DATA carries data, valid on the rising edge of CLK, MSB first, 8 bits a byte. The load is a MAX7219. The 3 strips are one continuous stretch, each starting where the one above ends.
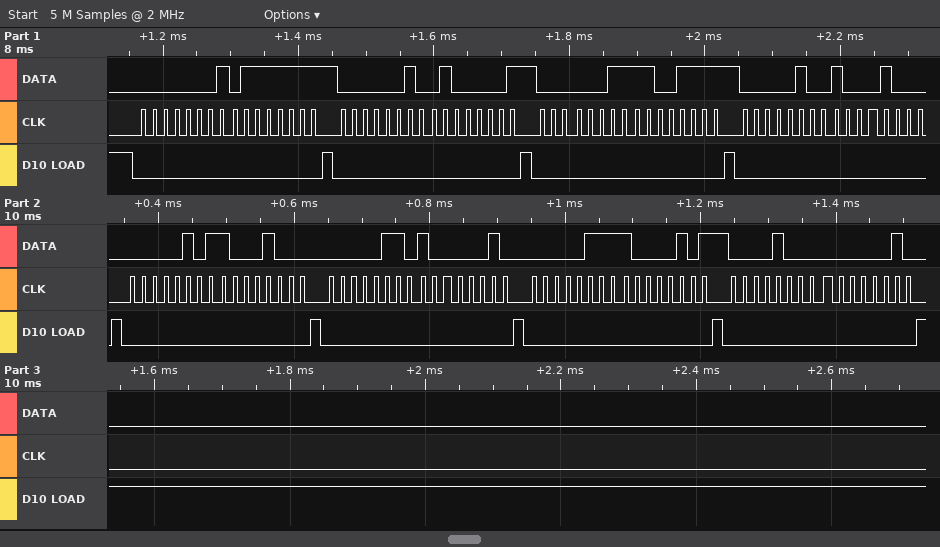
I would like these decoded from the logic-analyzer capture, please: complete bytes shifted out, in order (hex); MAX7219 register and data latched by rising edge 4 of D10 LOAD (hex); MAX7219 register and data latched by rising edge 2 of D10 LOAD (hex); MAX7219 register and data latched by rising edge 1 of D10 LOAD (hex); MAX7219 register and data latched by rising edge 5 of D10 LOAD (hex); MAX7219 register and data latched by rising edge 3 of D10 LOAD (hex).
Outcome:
0x01 0x7F 0x02 0x41 0x03 0xCF 0x04 0x88 0x05 0x88 0x06 0x82 0x07 0x85 0x08 0x02
register 0x4, data 0x88
register 0x2, data 0x41
register 0x1, data 0x7F
register 0x5, data 0x88
register 0x3, data 0xCF
